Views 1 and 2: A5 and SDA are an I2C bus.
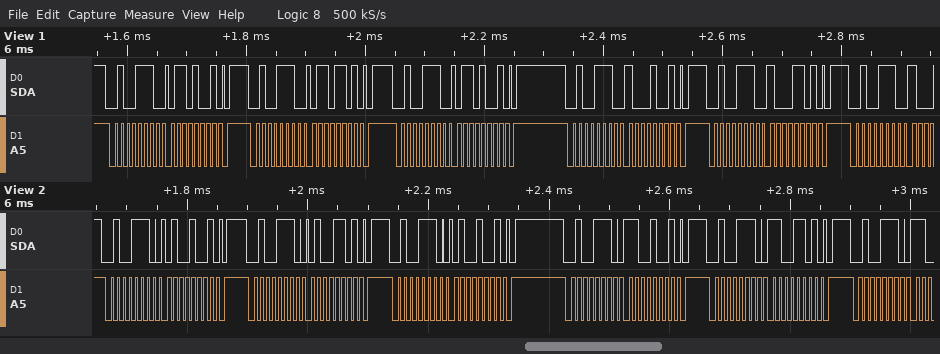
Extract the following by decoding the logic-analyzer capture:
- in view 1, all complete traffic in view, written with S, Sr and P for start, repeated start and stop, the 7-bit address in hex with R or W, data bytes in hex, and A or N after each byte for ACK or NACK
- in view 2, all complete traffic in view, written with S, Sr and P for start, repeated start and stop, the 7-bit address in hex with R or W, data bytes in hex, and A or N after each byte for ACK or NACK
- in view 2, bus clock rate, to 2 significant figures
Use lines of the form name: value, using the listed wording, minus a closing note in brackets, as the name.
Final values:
in view 1, all complete traffic in view, written with S, Sr and P for start, repeated start and stop, the 7-bit address in hex with R or W, data bytes in hex, and A or N after each byte for ACK or NACK: S 27W A 69 A P S 27W A 6D A P S 27W A 69 A P S 27W A 89 A P S 27W A 8D A P S 27W A
in view 2, all complete traffic in view, written with S, Sr and P for start, repeated start and stop, the 7-bit address in hex with R or W, data bytes in hex, and A or N after each byte for ACK or NACK: S 27W A 49 A P S 27W A 4D A P S 27W A 49 A P S 27W A C9 A P S 27W A CD A P S 27W A
in view 2, bus clock rate, to 2 significant figures: 100 kHz
